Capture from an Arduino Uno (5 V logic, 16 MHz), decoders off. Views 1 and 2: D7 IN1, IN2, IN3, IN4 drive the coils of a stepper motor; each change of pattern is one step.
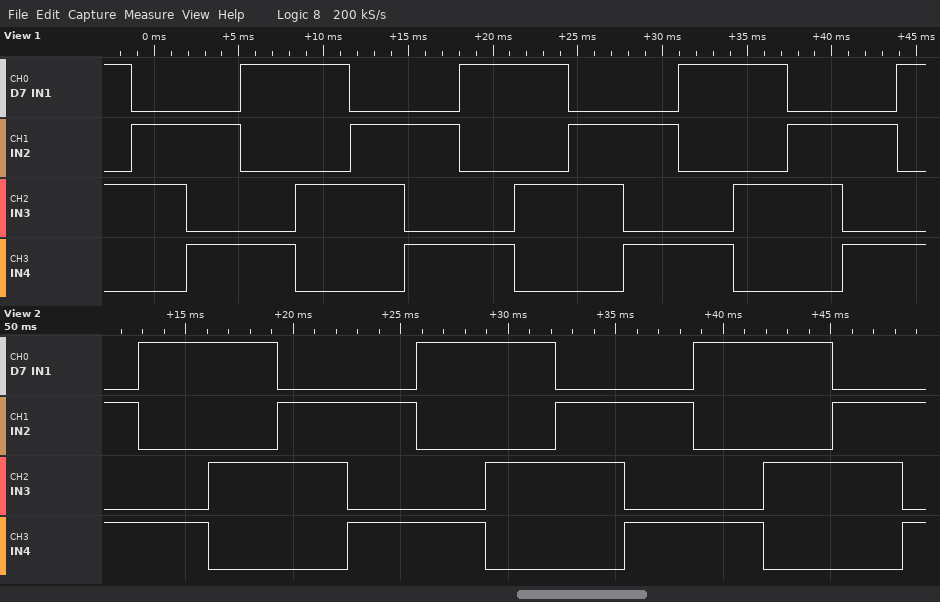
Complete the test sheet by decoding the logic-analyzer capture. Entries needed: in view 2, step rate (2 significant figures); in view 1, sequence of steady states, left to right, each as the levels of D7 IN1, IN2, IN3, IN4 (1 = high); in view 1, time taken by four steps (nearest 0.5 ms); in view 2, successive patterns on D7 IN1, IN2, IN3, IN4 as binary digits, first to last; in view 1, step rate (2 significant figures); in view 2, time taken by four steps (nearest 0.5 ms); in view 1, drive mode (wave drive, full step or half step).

310 steps/s
1010 0110 0101 1001 1010 0110 0101 1001 1010 0110 0101 1001 1010 0110 0101 1001
13.0 ms
0101 1001 1010 0110 0101 1001 1010 0110 0101 1001 1010 0110 0101
310 steps/s
13.0 ms
full step
